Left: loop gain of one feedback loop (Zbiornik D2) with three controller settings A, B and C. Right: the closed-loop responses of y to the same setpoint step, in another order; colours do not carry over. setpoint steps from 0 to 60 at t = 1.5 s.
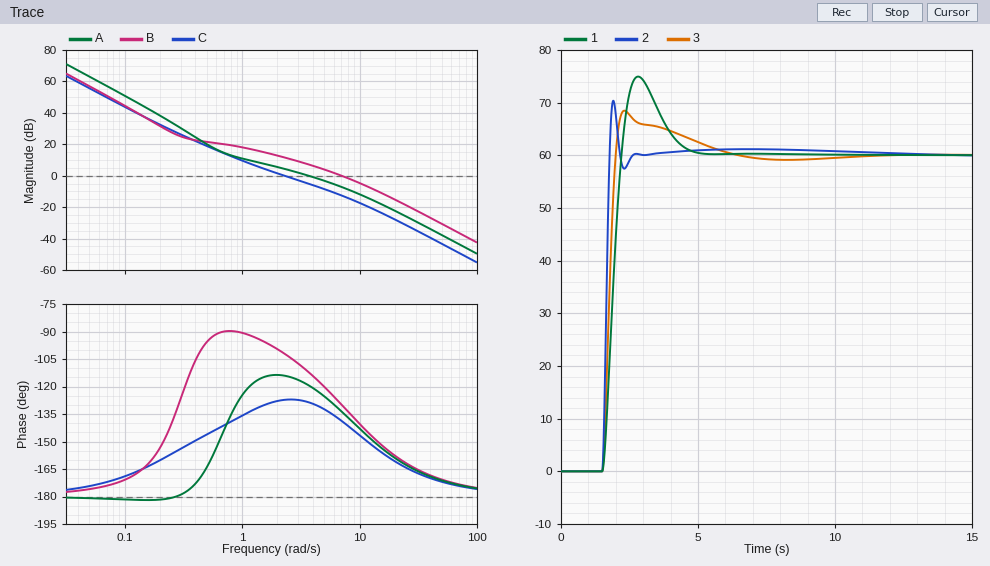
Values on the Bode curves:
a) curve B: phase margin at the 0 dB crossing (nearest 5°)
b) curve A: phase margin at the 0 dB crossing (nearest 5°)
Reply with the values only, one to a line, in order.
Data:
50°
60°
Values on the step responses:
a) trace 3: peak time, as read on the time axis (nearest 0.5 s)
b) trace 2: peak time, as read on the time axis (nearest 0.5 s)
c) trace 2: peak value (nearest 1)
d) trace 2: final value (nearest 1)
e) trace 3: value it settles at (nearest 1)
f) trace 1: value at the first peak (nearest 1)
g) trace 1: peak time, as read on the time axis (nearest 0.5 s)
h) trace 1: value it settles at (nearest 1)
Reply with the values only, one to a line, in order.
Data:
2.5 s
2.0 s
70
60
60
75
3.0 s
60
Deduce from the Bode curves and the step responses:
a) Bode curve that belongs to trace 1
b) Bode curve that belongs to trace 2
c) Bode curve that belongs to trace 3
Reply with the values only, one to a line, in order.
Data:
C
B
A
